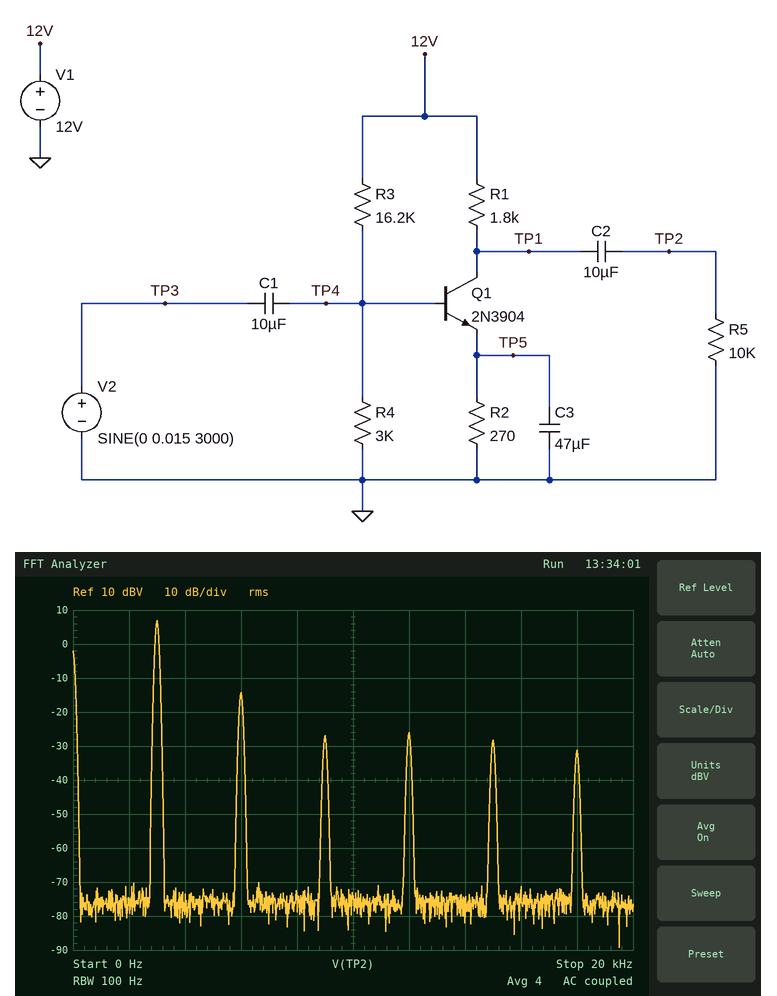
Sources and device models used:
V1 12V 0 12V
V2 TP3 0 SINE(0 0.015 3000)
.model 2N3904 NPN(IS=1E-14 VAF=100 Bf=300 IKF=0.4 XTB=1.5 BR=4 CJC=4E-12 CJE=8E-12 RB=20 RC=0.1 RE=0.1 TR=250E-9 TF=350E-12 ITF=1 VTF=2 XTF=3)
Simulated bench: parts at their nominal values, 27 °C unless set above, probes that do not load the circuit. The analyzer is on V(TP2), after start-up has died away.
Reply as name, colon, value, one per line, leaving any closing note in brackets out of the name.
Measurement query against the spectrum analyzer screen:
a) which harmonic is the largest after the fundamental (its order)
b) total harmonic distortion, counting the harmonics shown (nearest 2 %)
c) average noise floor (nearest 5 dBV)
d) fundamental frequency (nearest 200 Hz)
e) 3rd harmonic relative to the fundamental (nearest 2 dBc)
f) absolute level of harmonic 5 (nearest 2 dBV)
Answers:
which harmonic is the largest after the fundamental: 2
total harmonic distortion, counting the harmonics shown: 10 %
average noise floor: -75 dBV
fundamental frequency: 3.0 kHz
3rd harmonic relative to the fundamental: -34 dBc
absolute level of harmonic 5: -28 dBV
